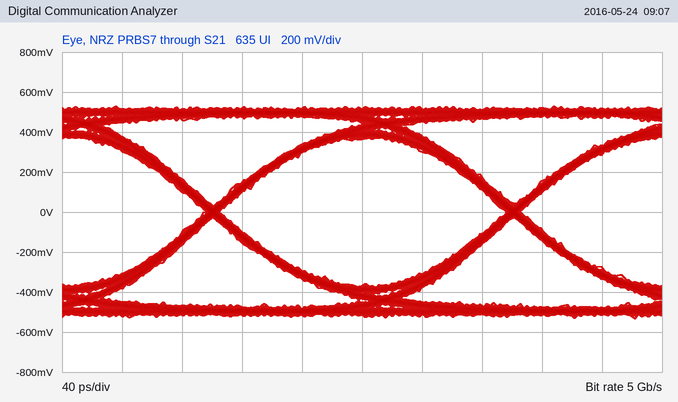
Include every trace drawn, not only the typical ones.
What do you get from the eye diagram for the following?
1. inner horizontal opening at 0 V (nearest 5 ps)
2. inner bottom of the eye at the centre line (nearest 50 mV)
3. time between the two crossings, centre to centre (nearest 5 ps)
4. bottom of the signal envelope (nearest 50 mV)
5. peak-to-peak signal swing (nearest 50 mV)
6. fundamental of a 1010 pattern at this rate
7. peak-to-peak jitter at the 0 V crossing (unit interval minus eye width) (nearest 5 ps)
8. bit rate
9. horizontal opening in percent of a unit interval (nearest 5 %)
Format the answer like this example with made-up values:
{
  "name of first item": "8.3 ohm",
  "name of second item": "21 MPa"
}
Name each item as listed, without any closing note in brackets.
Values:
{
  "inner horizontal opening at 0 V": "190 ps",
  "inner bottom of the eye at the centre line": "-350 mV",
  "time between the two crossings, centre to centre": "200 ps",
  "bottom of the signal envelope": "-550 mV",
  "peak-to-peak signal swing": "1.05 V",
  "fundamental of a 1010 pattern at this rate": "2.5 GHz",
  "peak-to-peak jitter at the 0 V crossing (unit interval minus eye width)": "10 ps",
  "bit rate": "5 Gb/s",
  "horizontal opening in percent of a unit interval": "95 %"
}
